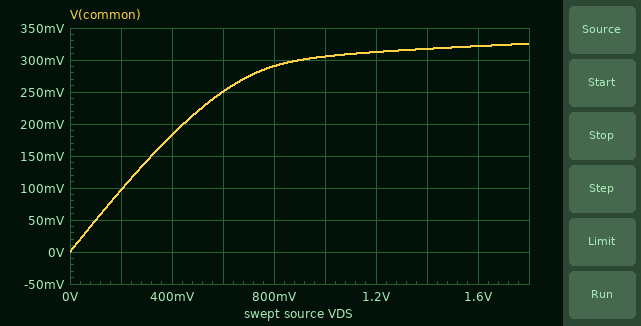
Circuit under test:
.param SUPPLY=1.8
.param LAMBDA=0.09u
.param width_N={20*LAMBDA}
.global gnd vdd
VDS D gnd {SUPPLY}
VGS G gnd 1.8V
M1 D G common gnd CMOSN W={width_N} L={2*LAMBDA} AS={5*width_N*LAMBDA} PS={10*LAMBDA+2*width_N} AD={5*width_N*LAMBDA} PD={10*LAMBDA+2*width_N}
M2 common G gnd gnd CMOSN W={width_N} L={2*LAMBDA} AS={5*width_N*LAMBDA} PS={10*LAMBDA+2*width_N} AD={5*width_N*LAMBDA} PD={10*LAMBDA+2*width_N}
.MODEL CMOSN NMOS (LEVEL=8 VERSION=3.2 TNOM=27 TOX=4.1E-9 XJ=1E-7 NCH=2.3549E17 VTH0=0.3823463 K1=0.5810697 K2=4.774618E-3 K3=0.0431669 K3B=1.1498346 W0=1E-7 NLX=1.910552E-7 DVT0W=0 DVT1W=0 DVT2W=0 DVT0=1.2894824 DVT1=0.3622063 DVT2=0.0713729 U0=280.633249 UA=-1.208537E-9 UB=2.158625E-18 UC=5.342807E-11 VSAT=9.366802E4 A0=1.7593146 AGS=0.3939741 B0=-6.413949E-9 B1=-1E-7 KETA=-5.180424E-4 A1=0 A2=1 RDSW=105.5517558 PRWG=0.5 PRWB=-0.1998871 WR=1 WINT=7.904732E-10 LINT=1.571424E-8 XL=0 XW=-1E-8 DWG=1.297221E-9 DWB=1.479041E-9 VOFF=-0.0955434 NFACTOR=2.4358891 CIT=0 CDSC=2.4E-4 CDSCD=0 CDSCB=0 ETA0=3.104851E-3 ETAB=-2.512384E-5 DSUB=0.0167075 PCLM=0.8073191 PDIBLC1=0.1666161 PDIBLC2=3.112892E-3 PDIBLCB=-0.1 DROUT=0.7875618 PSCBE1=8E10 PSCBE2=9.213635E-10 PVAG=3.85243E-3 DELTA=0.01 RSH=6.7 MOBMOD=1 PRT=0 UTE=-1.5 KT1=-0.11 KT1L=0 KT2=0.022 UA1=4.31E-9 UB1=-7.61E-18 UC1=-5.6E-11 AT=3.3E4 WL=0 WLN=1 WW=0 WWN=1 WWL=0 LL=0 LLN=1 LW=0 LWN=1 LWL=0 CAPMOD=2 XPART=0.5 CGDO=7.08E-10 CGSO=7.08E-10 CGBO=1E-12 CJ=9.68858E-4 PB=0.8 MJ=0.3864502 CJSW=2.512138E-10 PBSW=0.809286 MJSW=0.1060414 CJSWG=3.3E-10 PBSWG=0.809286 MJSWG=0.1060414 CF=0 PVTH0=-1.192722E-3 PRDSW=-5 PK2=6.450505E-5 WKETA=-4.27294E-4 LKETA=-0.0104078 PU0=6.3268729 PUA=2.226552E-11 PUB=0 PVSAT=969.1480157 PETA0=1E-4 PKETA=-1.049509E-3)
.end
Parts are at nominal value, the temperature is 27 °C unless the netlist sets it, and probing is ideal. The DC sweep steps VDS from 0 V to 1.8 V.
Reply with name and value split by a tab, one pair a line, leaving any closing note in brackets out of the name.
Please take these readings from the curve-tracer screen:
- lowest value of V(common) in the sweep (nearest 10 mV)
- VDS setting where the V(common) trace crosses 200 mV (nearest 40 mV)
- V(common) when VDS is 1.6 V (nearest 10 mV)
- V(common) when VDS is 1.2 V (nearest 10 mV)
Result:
lowest value of V(common) in the sweep	0 V
VDS setting where the V(common) trace crosses 200 mV	440 mV
V(common) when VDS is 1.6 V	320 mV
V(common) when VDS is 1.2 V	310 mV
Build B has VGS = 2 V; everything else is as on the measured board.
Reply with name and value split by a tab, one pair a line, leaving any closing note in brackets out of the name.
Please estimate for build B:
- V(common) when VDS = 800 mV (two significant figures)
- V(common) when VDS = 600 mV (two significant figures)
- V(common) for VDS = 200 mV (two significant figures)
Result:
V(common) when VDS = 800 mV	320 mV
V(common) when VDS = 600 mV	260 mV
V(common) for VDS = 200 mV	98 mV
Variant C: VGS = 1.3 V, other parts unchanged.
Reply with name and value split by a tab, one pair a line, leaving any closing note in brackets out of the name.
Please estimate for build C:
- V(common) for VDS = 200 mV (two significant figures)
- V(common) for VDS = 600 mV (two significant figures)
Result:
V(common) for VDS = 200 mV	92 mV
V(common) for VDS = 600 mV	190 mV
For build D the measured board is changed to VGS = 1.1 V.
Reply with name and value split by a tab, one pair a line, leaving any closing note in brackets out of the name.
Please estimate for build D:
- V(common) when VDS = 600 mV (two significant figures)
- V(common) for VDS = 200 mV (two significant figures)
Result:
V(common) when VDS = 600 mV	150 mV
V(common) for VDS = 200 mV	88 mV
